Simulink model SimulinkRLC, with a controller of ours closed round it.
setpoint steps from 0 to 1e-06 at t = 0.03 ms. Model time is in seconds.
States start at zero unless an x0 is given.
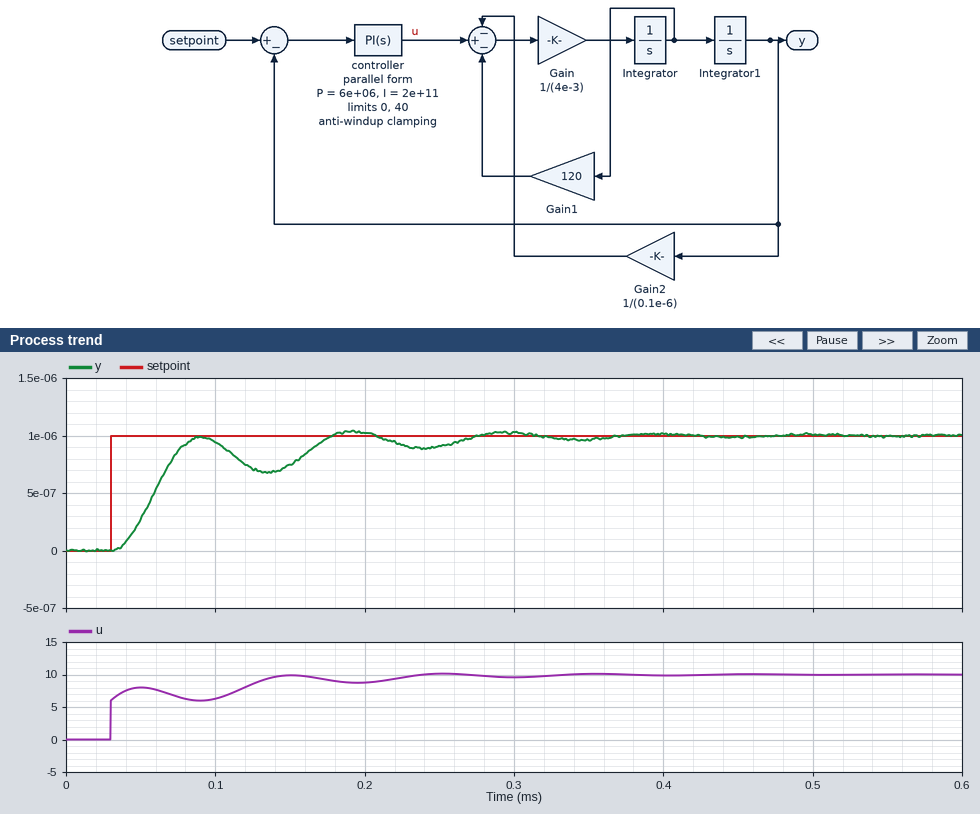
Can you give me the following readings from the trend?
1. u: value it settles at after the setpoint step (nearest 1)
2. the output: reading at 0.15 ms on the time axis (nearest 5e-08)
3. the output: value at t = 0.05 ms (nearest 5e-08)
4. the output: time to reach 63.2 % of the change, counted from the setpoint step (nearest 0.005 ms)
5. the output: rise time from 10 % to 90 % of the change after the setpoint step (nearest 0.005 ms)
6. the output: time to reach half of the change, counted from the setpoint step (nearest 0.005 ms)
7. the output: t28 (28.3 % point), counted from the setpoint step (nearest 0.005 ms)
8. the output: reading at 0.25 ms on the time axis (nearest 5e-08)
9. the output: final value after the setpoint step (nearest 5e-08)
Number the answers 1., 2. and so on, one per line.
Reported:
1. 10
2. 0.00000075
3. 0.00000025
4. 0.035 ms
5. 0.035 ms
6. 0.030 ms
7. 0.020 ms
8. 0.00000090
9. 0.00000100
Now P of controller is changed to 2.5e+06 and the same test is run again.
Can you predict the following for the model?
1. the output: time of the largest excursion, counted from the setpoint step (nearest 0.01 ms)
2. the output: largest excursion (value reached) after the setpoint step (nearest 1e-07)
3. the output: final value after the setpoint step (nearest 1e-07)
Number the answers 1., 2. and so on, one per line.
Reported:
1. 0.19 ms
2. 0.0000011
3. 0.0000010
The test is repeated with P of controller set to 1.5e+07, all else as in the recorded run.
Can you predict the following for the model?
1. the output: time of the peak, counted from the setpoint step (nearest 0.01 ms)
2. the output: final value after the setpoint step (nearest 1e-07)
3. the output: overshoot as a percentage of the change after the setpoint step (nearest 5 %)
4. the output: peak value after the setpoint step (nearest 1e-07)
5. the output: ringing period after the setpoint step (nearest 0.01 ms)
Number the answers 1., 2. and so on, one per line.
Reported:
1. 0.04 ms
2. 0.0000010
3. 10 %
4. 0.0000011
5. 0.08 ms
